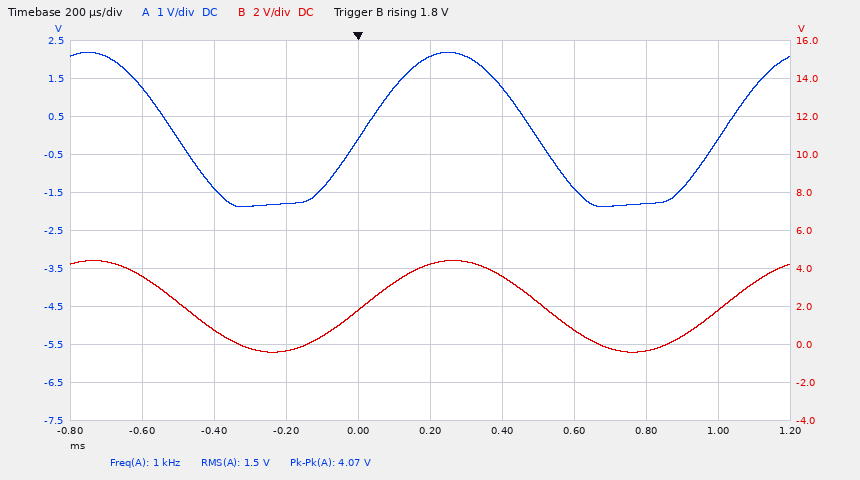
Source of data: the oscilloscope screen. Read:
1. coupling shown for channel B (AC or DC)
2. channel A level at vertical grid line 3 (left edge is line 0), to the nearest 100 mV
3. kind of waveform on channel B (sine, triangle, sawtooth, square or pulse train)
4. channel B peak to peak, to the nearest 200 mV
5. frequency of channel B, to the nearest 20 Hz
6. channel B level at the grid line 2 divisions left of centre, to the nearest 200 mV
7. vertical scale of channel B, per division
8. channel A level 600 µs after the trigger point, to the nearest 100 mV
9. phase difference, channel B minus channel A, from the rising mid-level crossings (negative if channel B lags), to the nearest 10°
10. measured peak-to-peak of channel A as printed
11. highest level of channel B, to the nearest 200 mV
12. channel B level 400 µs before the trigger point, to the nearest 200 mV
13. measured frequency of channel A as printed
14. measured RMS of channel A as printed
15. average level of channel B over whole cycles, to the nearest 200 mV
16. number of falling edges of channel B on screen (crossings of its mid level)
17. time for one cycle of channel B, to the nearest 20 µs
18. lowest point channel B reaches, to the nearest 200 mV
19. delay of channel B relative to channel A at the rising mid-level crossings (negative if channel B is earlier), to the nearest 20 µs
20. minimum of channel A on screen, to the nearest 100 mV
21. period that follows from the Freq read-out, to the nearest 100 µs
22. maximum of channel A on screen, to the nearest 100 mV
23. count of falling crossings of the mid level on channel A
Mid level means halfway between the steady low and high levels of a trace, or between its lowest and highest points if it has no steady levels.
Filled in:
DC
-1.8 V
sine
4.8 V
1.00 kHz
-400 mV
2 V
-1.4 V
0°
4.07 V
4.4 V
800 mV
1 kHz
1.5 V
2.0 V
2
1.00 ms
-400 mV
0 µs
-1.9 V
1.0 ms
2.2 V
2
